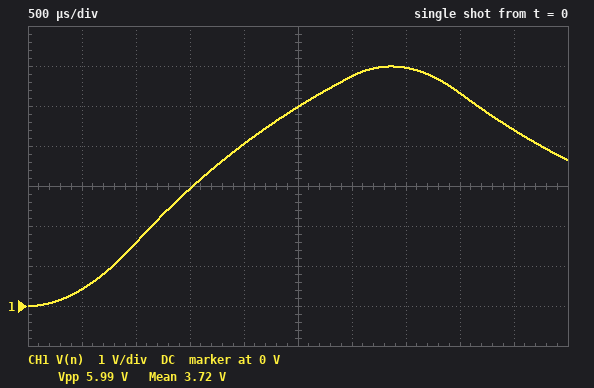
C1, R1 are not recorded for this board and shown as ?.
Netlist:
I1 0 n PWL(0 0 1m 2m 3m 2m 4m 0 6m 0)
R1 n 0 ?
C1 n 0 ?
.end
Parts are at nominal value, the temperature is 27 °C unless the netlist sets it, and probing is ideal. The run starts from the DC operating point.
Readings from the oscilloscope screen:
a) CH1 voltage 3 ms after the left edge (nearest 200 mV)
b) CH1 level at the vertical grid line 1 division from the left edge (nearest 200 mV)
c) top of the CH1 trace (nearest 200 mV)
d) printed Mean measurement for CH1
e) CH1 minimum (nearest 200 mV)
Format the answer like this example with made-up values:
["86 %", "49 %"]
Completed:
["5.8 V", "400 mV", "6.0 V", "3.72 V", "0 V"]
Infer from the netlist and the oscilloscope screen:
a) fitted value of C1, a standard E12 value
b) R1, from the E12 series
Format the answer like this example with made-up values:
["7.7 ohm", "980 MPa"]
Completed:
["560 nF", "4.7 kΩ"]
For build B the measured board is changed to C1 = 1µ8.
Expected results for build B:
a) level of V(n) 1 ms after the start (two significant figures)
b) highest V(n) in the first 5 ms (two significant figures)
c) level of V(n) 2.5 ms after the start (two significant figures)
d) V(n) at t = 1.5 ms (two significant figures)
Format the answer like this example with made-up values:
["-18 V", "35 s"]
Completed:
["530 mV", "2.7 V", "2.0 V", "1.0 V"]
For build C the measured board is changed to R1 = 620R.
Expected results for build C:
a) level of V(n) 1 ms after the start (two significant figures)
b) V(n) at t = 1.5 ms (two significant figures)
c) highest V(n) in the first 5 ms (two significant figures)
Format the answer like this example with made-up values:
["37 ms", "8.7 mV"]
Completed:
["830 mV", "1.1 V", "1.2 V"]
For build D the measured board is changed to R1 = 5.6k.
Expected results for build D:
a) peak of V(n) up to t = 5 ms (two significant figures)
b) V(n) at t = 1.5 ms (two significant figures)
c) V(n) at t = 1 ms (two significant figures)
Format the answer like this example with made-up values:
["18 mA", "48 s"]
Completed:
["6.5 V", "3.0 V", "1.6 V"]
